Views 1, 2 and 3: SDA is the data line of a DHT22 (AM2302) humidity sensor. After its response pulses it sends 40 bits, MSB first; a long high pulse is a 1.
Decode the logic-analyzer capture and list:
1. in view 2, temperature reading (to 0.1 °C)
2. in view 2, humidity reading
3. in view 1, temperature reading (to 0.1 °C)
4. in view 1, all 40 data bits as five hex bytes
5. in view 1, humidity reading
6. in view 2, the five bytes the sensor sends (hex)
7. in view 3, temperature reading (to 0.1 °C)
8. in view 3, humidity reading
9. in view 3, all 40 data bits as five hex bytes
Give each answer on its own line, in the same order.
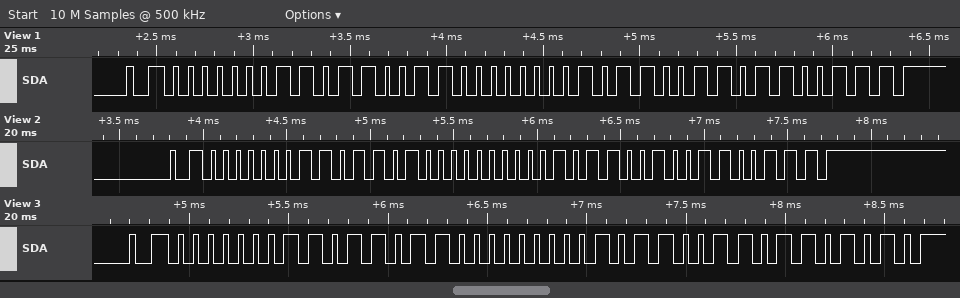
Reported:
17.8 °C
43.6 %
17.9 °C
01 B3 00 B3 67
43.5 %
01 B4 00 B2 67
17.9 °C
43.8 %
01 B6 00 B3 6A
